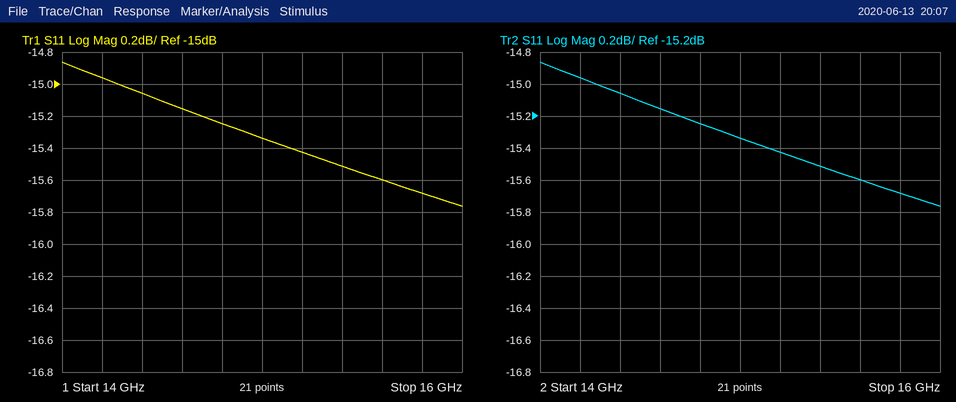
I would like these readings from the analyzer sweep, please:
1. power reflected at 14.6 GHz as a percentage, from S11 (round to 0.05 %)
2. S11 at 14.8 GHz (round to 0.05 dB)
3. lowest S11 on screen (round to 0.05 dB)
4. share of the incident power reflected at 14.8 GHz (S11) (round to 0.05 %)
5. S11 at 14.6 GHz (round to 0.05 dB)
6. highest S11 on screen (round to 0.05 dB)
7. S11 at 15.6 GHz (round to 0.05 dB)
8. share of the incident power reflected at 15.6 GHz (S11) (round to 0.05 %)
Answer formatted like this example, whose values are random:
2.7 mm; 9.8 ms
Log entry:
3.05 %; -15.25 dB; -15.75 dB; 3.00 %; -15.15 dB; -14.85 dB; -15.60 dB; 2.75 %
